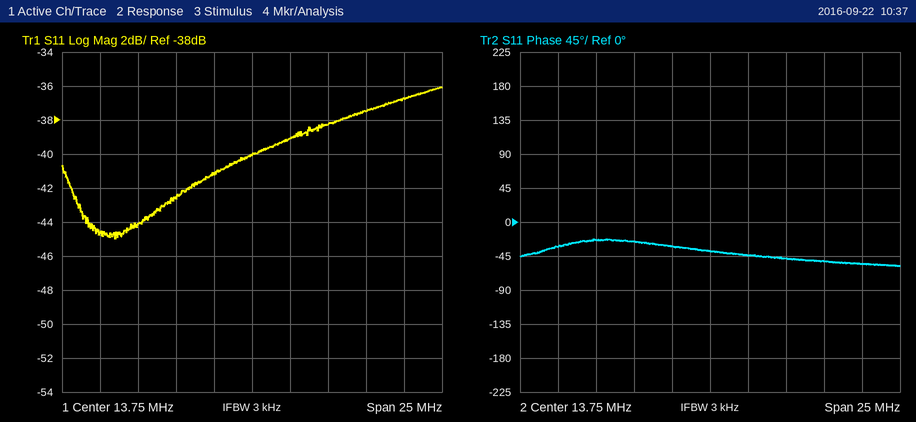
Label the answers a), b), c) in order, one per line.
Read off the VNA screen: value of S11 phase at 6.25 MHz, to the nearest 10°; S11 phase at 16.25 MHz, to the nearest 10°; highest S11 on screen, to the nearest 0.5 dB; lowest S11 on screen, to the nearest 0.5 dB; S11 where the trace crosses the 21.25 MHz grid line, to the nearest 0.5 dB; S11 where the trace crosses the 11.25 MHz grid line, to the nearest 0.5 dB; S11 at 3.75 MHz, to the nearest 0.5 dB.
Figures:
a) -20°
b) -40°
c) -36.0 dB
d) -45.0 dB
e) -37.5 dB
f) -41.0 dB
g) -44.5 dB
